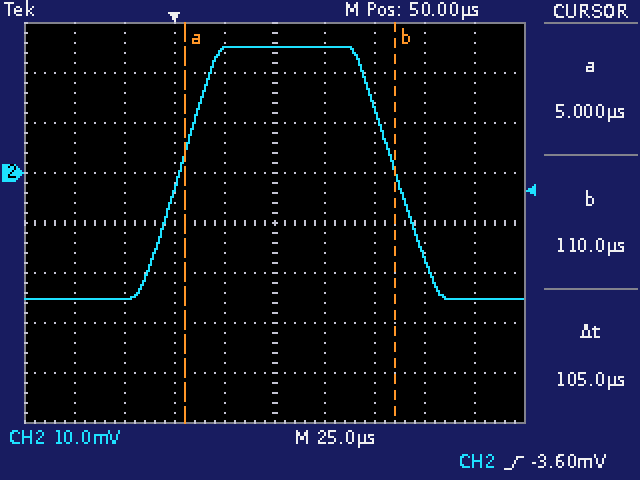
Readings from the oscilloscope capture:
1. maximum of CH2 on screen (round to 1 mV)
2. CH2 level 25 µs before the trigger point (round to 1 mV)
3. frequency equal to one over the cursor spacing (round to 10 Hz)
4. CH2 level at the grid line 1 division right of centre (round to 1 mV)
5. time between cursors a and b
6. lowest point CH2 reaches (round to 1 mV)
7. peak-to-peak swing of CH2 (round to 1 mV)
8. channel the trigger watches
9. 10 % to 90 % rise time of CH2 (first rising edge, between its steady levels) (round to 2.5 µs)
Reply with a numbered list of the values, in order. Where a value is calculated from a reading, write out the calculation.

1. 25 mV
2. -25 mV
3. 1 / 105 µs ≈ 9.52 kHz
4. 25 mV
5. 105 µs
6. -25 mV
7. 25 mV − (-25 mV) = 50 mV
8. CH2
9. 32.5 µs
